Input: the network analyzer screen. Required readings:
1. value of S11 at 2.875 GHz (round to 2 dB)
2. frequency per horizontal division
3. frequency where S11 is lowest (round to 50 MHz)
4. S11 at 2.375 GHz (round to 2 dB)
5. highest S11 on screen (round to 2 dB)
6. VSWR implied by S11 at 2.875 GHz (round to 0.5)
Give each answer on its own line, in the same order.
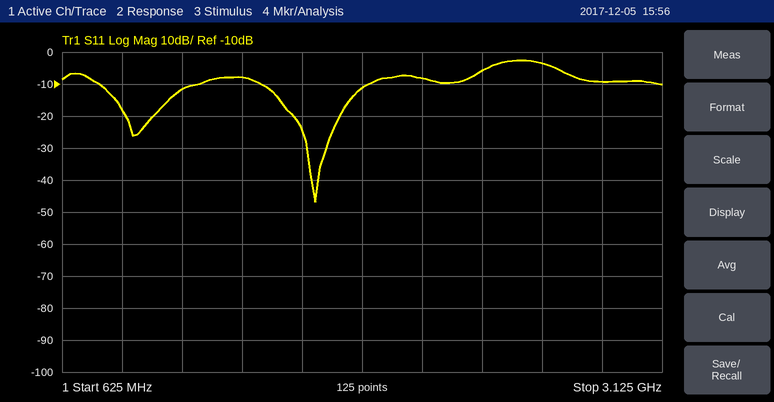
-10 dB
250 MHz
1.70 GHz
-6 dB
-2 dB
2.0
